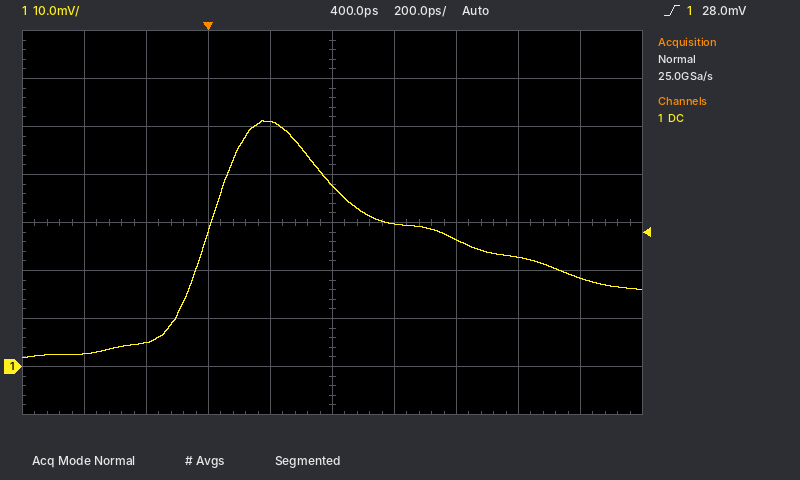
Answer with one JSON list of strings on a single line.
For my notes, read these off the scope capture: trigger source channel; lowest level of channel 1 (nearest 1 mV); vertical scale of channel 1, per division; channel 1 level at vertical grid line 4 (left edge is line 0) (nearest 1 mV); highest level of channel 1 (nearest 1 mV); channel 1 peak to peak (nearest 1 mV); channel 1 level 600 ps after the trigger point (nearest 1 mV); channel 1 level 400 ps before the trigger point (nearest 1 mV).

["channel 1", "2 mV", "10 mV", "51 mV", "51 mV", "49 mV", "30 mV", "3 mV"]
